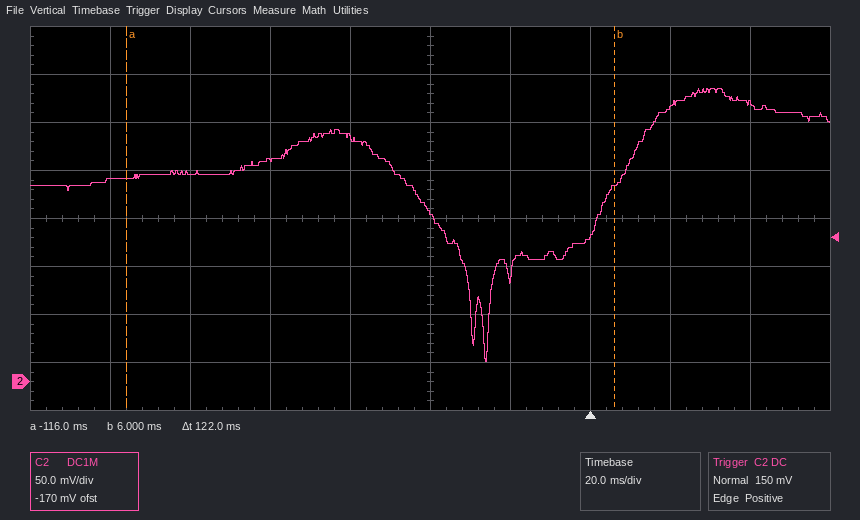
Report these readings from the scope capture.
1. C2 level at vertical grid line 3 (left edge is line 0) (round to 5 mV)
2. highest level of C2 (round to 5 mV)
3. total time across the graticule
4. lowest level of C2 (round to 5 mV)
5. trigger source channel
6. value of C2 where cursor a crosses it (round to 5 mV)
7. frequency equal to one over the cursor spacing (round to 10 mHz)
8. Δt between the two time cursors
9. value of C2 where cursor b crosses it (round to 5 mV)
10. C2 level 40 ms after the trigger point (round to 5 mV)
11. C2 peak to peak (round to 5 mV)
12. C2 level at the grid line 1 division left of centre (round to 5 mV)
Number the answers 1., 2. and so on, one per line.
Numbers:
1. 230 mV
2. 305 mV
3. 200 ms
4. 20 mV
5. C2
6. 210 mV
7. 8.20 Hz
8. 122 ms
9. 205 mV
10. 290 mV
11. 285 mV
12. 255 mV
